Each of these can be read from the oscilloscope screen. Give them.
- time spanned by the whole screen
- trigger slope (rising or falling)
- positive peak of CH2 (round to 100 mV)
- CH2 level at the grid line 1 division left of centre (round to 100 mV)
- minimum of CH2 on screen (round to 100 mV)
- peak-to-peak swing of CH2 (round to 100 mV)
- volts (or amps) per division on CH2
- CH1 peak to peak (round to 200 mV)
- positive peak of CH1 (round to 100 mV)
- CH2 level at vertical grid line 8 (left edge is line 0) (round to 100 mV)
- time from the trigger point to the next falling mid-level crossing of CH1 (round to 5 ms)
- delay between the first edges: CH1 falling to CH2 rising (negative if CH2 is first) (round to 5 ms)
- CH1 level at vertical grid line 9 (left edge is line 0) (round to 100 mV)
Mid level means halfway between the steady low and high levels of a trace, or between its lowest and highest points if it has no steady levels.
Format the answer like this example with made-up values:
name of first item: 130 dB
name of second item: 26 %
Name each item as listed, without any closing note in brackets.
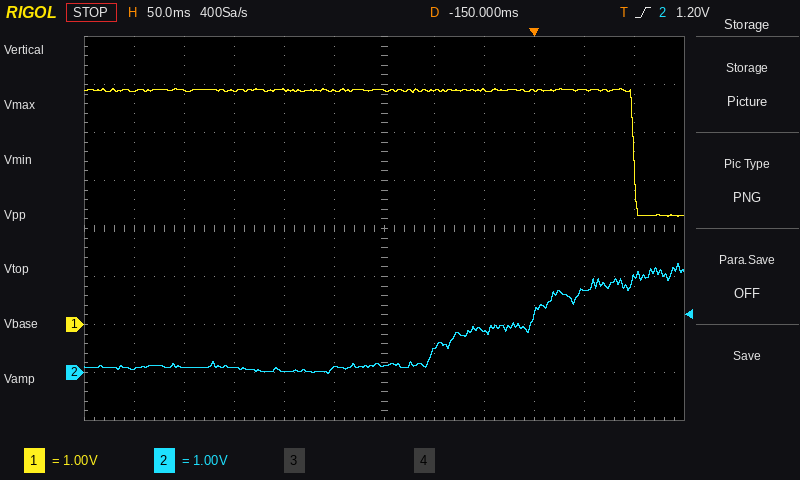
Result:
time spanned by the whole screen: 600 ms
trigger slope: rising
positive peak of CH2: 2.3 V
CH2 level at the grid line 1 division left of centre: 100 mV
minimum of CH2 on screen: 0.0 V
peak-to-peak swing of CH2: 2.3 V
volts (or amps) per division on CH2: 1 V
CH1 peak to peak: 2.6 V
positive peak of CH1: 4.9 V
CH2 level at vertical grid line 8 (left edge is line 0): 900 mV
time from the trigger point to the next falling mid-level crossing of CH1: 100 ms
delay between the first edges: CH1 falling to CH2 rising (negative if CH2 is first): -100 ms
CH1 level at vertical grid line 9 (left edge is line 0): 4.9 V
